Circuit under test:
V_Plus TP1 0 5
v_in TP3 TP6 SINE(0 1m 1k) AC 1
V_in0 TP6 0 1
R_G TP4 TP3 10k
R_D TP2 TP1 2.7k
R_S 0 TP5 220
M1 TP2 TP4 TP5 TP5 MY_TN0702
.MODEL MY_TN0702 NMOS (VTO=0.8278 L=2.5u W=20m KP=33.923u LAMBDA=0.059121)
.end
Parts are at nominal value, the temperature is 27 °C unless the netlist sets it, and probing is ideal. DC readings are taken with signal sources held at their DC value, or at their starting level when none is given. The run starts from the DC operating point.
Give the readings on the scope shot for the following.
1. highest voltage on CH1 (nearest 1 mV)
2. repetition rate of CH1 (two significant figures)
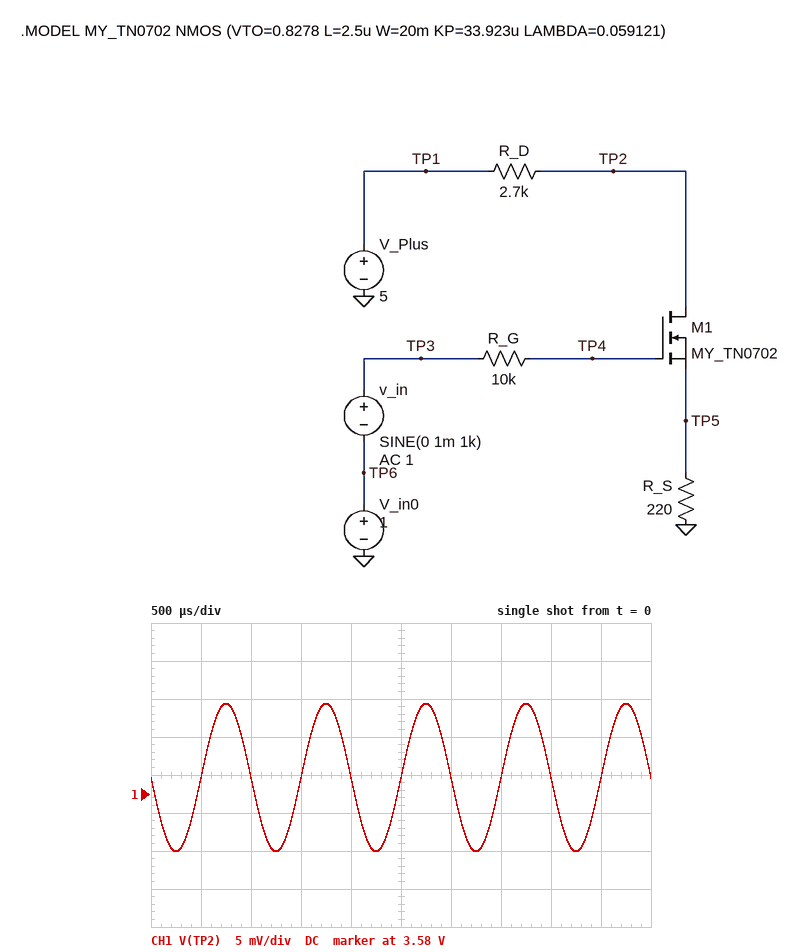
3.592 V
1.0 kHz
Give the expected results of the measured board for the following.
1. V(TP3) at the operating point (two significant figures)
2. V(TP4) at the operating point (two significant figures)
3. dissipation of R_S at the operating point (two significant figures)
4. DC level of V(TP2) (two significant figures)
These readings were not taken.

1.0 V
1.0 V
61 µW
3.6 V
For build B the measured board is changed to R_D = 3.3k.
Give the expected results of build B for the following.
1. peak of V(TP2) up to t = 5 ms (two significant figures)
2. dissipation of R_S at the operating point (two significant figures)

3.3 V
60 µW
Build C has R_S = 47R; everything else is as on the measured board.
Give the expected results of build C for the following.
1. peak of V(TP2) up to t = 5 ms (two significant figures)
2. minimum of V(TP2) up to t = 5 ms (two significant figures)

1.0 V
940 mV
